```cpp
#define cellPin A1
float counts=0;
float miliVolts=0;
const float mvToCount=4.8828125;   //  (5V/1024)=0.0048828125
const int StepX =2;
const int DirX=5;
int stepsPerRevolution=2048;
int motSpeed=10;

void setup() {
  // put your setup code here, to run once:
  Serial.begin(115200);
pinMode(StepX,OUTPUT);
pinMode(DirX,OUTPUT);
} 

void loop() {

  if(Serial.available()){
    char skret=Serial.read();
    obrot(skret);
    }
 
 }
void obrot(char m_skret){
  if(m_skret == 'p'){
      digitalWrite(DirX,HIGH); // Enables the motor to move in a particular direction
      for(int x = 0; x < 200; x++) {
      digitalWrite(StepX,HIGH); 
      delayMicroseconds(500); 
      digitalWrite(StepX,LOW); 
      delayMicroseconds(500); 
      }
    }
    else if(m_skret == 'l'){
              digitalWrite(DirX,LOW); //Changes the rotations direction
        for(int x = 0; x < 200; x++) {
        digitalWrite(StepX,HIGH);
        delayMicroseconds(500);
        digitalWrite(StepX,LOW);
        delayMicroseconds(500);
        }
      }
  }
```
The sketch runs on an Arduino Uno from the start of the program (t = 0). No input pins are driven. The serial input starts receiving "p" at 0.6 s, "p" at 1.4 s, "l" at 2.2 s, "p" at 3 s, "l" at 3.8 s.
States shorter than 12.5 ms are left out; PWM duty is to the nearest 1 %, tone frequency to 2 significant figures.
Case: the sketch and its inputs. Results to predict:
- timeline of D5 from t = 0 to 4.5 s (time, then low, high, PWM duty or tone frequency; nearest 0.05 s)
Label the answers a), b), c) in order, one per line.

a) 0 s low; 0.6 s high; 2.2 s low; 3 s high; 3.8 s low
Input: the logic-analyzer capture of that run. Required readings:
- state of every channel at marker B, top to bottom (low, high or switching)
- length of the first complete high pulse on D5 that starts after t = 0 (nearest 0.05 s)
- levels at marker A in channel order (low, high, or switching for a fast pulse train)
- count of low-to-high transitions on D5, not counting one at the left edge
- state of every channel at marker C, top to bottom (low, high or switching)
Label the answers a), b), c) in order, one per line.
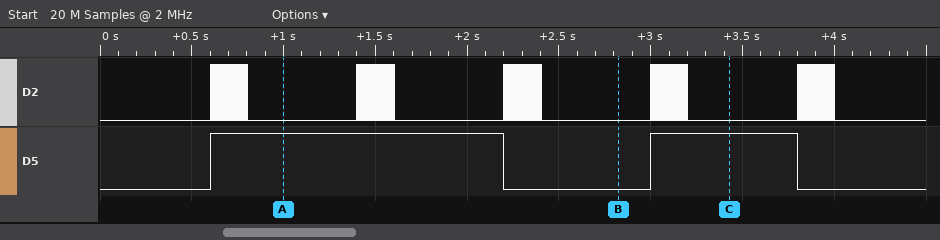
a) D2 low, D5 low
b) 1.60 s
c) D2 low, D5 high
d) 2
e) D2 low, D5 high
